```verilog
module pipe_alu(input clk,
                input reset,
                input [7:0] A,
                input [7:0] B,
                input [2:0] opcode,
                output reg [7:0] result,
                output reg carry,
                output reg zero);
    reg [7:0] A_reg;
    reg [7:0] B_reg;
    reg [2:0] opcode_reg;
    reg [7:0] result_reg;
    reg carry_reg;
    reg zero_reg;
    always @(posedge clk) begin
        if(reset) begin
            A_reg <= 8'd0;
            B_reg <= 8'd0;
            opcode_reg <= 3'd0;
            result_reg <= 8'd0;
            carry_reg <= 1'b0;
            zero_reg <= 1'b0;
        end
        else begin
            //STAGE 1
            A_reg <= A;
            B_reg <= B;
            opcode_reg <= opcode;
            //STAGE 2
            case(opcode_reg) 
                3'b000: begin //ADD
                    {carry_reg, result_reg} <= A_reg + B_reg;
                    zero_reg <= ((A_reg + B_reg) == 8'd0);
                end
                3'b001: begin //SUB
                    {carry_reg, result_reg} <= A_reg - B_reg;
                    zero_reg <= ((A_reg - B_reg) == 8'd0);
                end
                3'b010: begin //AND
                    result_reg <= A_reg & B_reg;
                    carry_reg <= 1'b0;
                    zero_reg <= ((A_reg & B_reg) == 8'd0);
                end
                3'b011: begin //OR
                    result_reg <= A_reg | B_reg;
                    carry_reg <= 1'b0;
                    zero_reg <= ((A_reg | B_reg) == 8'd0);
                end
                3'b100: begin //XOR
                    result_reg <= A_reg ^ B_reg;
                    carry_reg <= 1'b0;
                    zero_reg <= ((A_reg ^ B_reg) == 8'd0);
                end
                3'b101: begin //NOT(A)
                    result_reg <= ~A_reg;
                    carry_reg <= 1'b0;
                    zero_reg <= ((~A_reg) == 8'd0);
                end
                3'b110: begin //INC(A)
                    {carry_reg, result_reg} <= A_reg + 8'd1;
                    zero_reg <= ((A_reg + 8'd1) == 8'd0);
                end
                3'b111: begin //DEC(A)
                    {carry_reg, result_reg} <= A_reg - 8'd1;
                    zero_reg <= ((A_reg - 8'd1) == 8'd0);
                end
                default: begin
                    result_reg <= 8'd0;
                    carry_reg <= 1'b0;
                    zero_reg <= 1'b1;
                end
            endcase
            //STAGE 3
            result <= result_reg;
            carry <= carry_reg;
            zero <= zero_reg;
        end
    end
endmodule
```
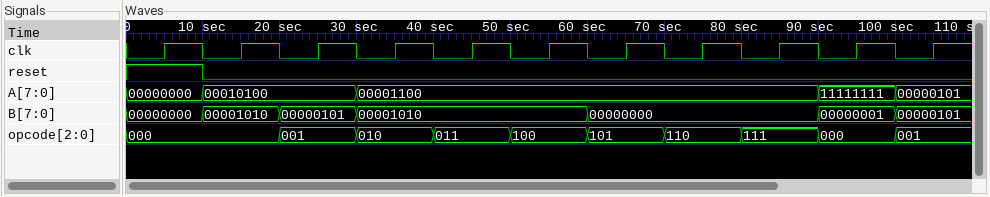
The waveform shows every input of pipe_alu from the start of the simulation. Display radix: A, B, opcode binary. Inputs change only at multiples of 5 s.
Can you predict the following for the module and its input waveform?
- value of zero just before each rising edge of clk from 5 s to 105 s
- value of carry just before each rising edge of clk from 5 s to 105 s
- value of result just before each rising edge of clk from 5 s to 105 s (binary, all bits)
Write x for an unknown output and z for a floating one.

x x 0 1 0 0 0 0 0 0 0
x x 0 0 0 0 0 0 0 0 0
x, x, 00000000, 00000000, 00011110, 00001111, 00001000, 00001110, 00000110, 11110011, 00001101
